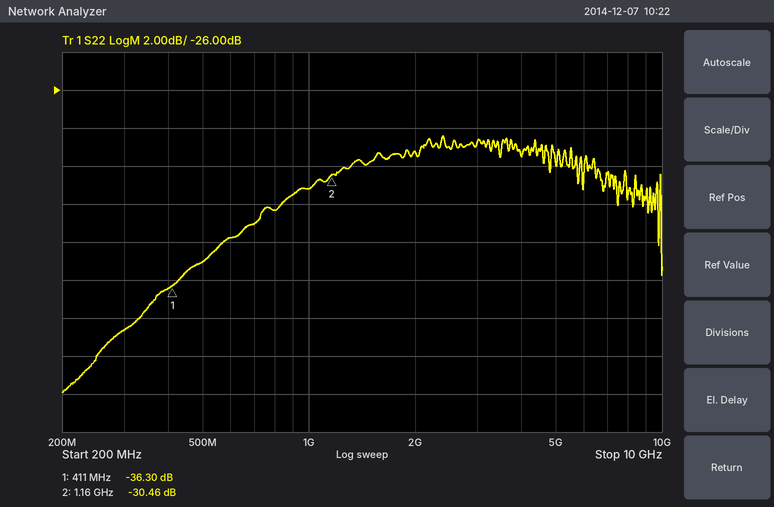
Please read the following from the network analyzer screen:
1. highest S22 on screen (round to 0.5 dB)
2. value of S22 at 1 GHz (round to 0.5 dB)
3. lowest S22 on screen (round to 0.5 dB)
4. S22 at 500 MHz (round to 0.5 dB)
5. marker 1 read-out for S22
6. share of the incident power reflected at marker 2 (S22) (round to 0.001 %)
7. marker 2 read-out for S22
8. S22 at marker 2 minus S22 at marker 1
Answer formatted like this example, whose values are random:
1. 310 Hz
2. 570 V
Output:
1. -28.5 dB
2. -31.0 dB
3. -42.0 dB
4. -35.0 dB
5. -36.30 dB
6. 0.090 %
7. -30.46 dB
8. 5.84 dB
